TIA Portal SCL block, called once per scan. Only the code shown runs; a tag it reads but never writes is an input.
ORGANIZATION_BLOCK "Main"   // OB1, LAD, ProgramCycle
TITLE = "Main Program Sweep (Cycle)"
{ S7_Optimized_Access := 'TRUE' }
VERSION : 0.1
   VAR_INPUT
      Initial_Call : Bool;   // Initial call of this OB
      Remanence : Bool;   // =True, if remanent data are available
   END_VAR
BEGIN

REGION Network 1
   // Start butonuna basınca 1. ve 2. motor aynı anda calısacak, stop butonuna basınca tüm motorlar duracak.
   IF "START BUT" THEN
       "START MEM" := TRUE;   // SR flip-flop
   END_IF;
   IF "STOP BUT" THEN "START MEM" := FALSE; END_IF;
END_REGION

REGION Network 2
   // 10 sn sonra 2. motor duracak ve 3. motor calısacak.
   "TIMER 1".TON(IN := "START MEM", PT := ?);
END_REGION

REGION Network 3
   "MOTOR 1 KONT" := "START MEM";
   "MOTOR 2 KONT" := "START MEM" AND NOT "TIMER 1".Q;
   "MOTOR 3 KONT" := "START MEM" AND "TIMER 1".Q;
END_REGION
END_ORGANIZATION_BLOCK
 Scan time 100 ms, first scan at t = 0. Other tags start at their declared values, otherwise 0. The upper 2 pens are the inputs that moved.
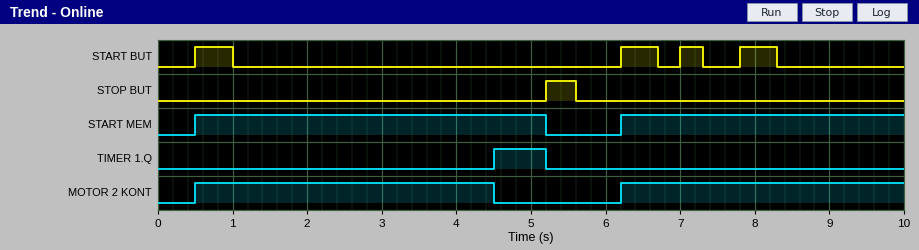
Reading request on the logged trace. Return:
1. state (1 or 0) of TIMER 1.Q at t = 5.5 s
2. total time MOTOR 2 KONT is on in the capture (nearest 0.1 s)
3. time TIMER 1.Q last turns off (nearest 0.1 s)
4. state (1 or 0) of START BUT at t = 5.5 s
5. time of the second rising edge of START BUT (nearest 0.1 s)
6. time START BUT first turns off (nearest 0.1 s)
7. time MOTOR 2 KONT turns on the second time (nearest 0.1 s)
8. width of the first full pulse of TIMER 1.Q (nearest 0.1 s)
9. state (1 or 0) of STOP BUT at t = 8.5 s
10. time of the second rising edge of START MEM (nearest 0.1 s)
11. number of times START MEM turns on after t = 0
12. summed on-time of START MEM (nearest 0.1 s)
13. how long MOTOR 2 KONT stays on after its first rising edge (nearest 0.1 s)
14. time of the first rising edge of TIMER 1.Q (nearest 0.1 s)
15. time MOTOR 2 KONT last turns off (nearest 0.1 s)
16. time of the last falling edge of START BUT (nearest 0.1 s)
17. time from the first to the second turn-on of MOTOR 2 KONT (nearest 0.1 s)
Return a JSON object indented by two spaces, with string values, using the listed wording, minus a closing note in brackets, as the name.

{
  "state (1 or 0) of TIMER 1.Q at t = 5.5 s": "0",
  "total time MOTOR 2 KONT is on in the capture": "7.8 s",
  "time TIMER 1.Q last turns off": "5.2 s",
  "state (1 or 0) of START BUT at t = 5.5 s": "0",
  "time of the second rising edge of START BUT": "6.2 s",
  "time START BUT first turns off": "1.0 s",
  "time MOTOR 2 KONT turns on the second time": "6.2 s",
  "width of the first full pulse of TIMER 1.Q": "0.7 s",
  "state (1 or 0) of STOP BUT at t = 8.5 s": "0",
  "time of the second rising edge of START MEM": "6.2 s",
  "number of times START MEM turns on after t = 0": "2",
  "summed on-time of START MEM": "8.5 s",
  "how long MOTOR 2 KONT stays on after its first rising edge": "4.0 s",
  "time of the first rising edge of TIMER 1.Q": "4.5 s",
  "time MOTOR 2 KONT last turns off": "4.5 s",
  "time of the last falling edge of START BUT": "8.3 s",
  "time from the first to the second turn-on of MOTOR 2 KONT": "5.7 s"
}
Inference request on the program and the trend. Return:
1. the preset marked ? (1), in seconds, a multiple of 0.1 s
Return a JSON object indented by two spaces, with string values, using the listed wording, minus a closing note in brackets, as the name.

{
  "the preset marked ? (1), in seconds, a multiple of 0.1 s": "4.0 s"
}
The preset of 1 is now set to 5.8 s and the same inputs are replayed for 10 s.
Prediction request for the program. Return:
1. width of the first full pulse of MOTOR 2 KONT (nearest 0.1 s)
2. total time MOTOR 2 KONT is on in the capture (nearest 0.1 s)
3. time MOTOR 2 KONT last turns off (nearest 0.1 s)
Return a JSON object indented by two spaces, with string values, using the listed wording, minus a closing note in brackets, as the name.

{
  "width of the first full pulse of MOTOR 2 KONT": "4.7 s",
  "total time MOTOR 2 KONT is on in the capture": "8.5 s",
  "time MOTOR 2 KONT last turns off": "5.2 s"
}
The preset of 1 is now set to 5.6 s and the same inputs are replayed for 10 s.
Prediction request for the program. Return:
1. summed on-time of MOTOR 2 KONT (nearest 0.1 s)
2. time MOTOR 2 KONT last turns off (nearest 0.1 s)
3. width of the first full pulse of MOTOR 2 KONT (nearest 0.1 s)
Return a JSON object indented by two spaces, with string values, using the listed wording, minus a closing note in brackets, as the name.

{
  "summed on-time of MOTOR 2 KONT": "8.5 s",
  "time MOTOR 2 KONT last turns off": "5.2 s",
  "width of the first full pulse of MOTOR 2 KONT": "4.7 s"
}
